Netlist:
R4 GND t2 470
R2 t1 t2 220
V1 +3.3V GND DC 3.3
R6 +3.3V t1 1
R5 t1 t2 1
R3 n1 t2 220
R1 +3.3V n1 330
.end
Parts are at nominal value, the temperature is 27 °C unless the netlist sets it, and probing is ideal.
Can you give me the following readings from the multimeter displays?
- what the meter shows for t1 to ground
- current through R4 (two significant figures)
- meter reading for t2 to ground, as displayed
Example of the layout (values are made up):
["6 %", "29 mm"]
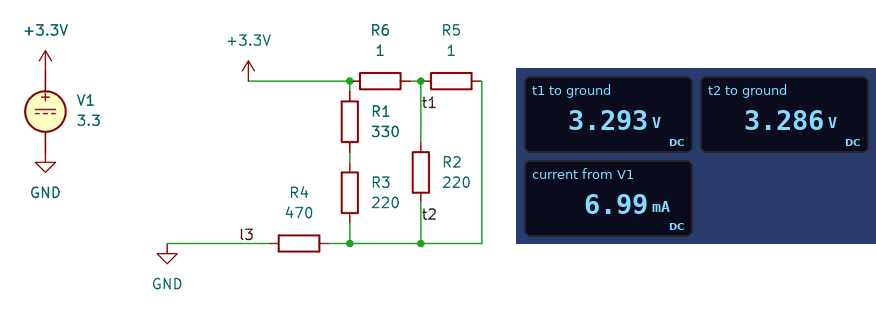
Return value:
["3.293 V", "7.0 mA", "3.286 V"]
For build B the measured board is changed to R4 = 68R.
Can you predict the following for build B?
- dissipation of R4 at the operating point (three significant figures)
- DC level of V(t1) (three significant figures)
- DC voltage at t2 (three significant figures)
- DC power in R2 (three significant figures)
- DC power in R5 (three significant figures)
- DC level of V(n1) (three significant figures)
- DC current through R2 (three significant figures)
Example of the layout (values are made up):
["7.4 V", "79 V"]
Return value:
["151 mW", "3.25 V", "3.21 V", "9.94 µW", "2.19 mW", "3.24 V", "213 µA"]
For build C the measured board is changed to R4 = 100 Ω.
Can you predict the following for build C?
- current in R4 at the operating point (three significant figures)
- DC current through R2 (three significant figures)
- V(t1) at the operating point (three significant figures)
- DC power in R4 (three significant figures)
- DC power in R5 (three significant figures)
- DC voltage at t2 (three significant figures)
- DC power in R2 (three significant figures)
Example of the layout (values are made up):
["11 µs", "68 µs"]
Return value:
["32.4 mA", "146 µA", "3.27 V", "105 mW", "1.03 mW", "3.24 V", "4.68 µW"]
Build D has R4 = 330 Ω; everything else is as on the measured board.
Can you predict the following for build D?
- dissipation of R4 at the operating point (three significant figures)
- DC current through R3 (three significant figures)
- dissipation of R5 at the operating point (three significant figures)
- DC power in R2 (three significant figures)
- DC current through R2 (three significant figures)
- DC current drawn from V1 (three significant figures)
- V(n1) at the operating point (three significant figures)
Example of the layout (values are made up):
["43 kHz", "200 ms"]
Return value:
["32.6 mW", "35.9 µA", "97.2 µW", "442 nW", "44.8 µA", "9.94 mA", "3.29 V"]
